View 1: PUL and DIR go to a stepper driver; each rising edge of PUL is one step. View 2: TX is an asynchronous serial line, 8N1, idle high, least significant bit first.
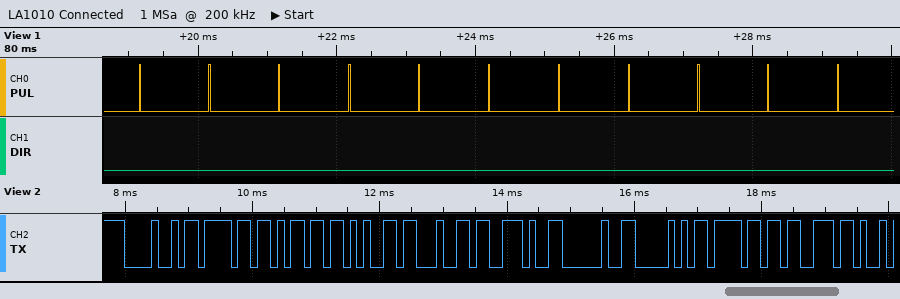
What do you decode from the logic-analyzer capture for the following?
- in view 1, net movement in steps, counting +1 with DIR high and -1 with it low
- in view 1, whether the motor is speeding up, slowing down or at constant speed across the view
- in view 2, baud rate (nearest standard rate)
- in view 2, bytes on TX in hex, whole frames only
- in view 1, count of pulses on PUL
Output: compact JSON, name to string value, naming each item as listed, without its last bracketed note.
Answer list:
{"in view 1, net movement in steps, counting +1 with DIR high and -1 with it low": "-11", "in view 1, whether the motor is speeding up, slowing down or at constant speed across the view": "constant speed", "in view 2, baud rate": "9600 baud", "in view 2, bytes on TX in hex, whole frames only": "48 6F 6D 65 64 2E 20 50 6F 73", "in view 1, count of pulses on PUL": "11"}
